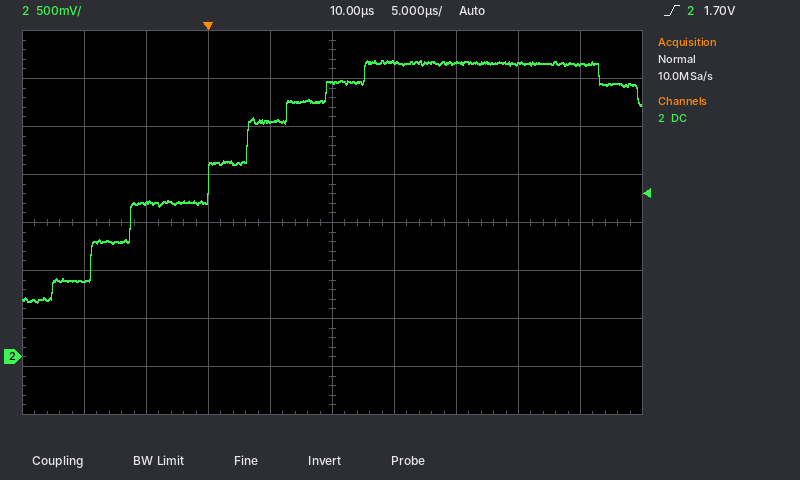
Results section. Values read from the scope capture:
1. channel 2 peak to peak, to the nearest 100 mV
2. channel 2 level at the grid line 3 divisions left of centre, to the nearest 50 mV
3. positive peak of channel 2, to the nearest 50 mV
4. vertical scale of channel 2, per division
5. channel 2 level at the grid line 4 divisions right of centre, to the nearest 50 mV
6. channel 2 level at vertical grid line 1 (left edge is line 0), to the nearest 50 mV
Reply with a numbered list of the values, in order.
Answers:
1. 2.50 V
2. 1.60 V
3. 3.10 V
4. 500 mV
5. 3.05 V
6. 800 mV
